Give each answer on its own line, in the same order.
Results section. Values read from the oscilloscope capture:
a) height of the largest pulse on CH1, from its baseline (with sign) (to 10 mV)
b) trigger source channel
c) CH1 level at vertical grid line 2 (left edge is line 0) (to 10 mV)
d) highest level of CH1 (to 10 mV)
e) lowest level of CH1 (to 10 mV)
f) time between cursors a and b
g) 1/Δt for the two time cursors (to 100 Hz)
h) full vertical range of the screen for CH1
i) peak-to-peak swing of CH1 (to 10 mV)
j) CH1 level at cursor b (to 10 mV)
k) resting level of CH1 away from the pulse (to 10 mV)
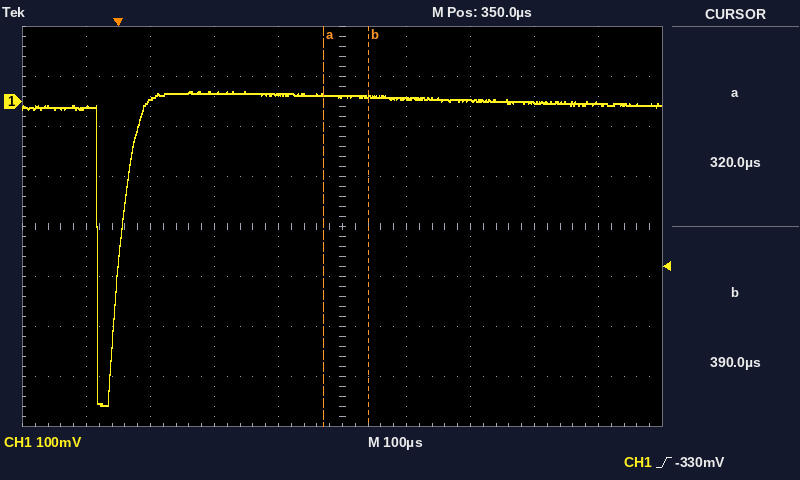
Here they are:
-610 mV
CH1
0 mV
20 mV
-610 mV
70 µs
14.3 kHz
800 mV
630 mV
10 mV
0 mV
